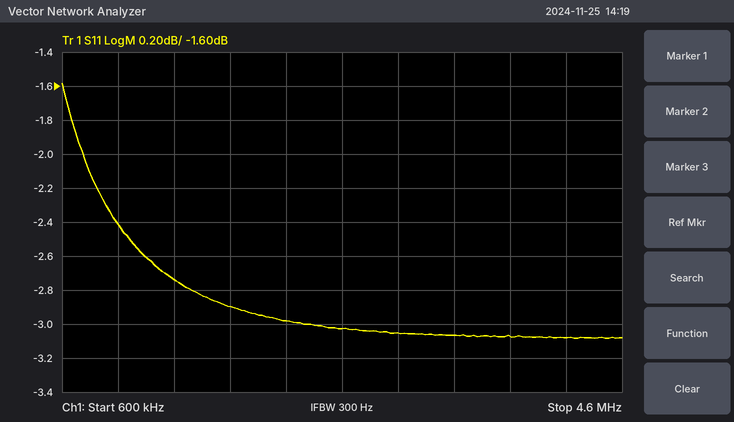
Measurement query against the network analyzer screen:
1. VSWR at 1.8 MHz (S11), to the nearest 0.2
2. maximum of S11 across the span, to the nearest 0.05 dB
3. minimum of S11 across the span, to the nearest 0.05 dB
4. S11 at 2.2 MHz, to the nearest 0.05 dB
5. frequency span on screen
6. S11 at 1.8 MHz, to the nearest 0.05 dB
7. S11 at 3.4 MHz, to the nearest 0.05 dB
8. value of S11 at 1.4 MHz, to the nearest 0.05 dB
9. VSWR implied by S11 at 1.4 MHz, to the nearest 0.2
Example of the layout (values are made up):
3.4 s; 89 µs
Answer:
6.0; -1.60 dB; -3.10 dB; -3.00 dB; 4 MHz; -2.90 dB; -3.05 dB; -2.75 dB; 6.4
